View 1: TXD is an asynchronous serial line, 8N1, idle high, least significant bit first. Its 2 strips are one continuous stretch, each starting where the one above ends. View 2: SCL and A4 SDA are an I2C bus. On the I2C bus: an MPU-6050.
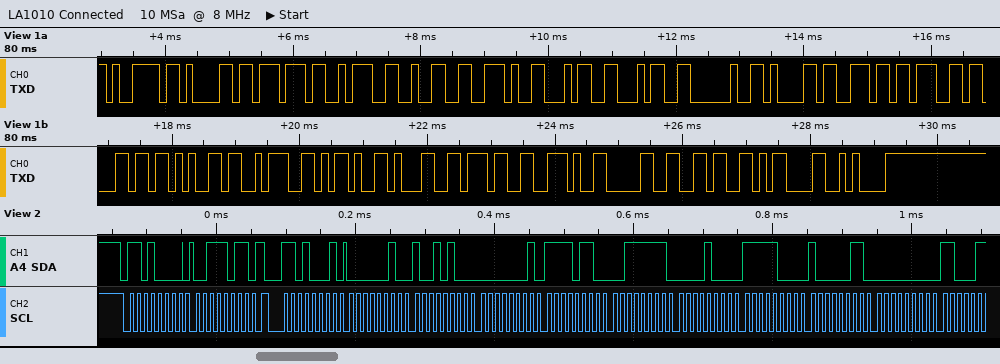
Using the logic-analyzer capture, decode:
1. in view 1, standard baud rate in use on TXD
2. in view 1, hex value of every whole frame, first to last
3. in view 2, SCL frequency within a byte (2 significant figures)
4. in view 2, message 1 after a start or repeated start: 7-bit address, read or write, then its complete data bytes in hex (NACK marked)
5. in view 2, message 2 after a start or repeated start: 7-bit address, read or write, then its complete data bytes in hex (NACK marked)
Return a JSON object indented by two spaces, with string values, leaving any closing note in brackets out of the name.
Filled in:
{
  "in view 1, standard baud rate in use on TXD": "9600 baud",
  "in view 1, hex value of every whole frame, first to last": "0x79 0x61 0x77 0x3A 0x32 0x2E 0x34 0x34 0x20 0x61 0x6E 0x67 0x6C 0x65 0x3A 0x2D 0x31 0x37 0x2E 0x30 0x36 0x0D 0x0A",
  "in view 2, SCL frequency within a byte": "100 kHz",
  "in view 2, message 1 after a start or repeated start: 7-bit address, read or write, then its complete data bytes in hex": "0x68 write: 3B",
  "in view 2, message 2 after a start or repeated start: 7-bit address, read or write, then its complete data bytes in hex": "0x68 read: 02 94 01 F6 3F 08 F8 83 00"
}
